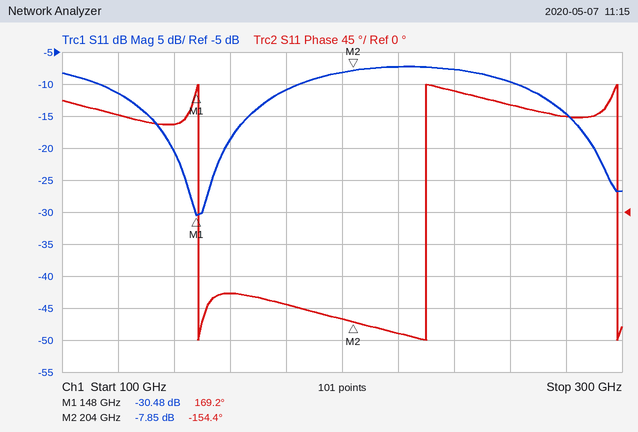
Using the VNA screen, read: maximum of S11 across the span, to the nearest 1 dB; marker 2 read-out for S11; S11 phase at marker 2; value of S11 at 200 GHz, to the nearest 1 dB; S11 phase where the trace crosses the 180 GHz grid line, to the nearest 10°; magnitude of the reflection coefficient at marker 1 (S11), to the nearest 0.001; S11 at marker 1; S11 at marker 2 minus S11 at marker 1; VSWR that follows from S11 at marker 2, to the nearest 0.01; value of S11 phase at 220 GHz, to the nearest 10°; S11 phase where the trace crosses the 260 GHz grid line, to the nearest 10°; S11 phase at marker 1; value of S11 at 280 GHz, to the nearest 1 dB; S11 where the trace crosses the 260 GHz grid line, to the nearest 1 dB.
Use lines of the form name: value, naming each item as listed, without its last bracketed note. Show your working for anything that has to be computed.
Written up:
maximum of S11 across the span, to the nearest 1 dB: -7 dB
marker 2 read-out for S11: -7.85 dB
S11 phase at marker 2: -154.4°
value of S11 at 200 GHz, to the nearest 1 dB: -8 dB
S11 phase where the trace crosses the 180 GHz grid line, to the nearest 10°: -130°
magnitude of the reflection coefficient at marker 1 (S11), to the nearest 0.001: 10^(-30.48/20) ≈ 0.030
S11 at marker 1: -30.48 dB
S11 at marker 2 minus S11 at marker 1: -7.85 − (-30.48) = 22.63 dB
VSWR that follows from S11 at marker 2, to the nearest 0.01: (1 + 0.4050)/(1 − 0.4050) ≈ 2.36
value of S11 phase at 220 GHz, to the nearest 10°: -170°
S11 phase where the trace crosses the 260 GHz grid line, to the nearest 10°: 150°
S11 phase at marker 1: 169.2°
value of S11 at 280 GHz, to the nearest 1 dB: -15 dB
S11 where the trace crosses the 260 GHz grid line, to the nearest 1 dB: -10 dB
